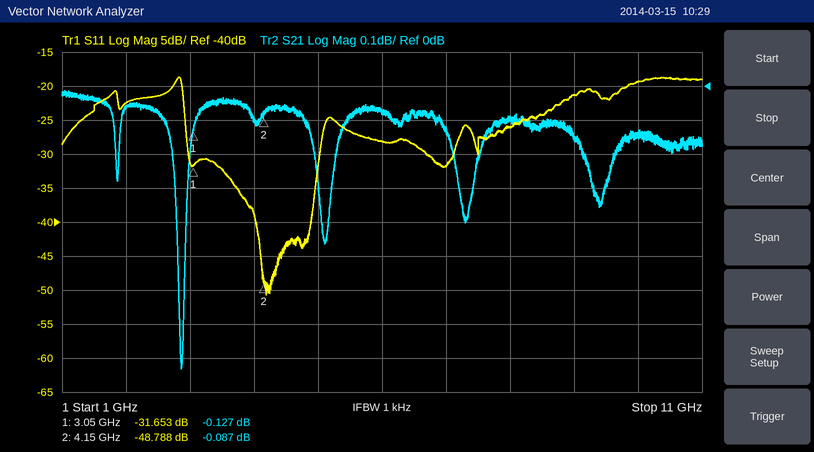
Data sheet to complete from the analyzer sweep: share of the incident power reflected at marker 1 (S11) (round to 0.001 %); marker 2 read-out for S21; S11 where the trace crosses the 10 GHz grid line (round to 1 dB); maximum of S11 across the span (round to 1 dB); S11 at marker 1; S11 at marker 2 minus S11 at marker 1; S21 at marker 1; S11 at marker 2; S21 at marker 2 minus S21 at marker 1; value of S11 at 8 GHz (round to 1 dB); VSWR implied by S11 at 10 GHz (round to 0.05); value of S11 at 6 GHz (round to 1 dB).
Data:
0.068 %
-0.087 dB
-19 dB
-19 dB
-31.653 dB
-17.135 dB
-0.127 dB
-48.788 dB
0.040 dB
-26 dB
1.25
-28 dB
